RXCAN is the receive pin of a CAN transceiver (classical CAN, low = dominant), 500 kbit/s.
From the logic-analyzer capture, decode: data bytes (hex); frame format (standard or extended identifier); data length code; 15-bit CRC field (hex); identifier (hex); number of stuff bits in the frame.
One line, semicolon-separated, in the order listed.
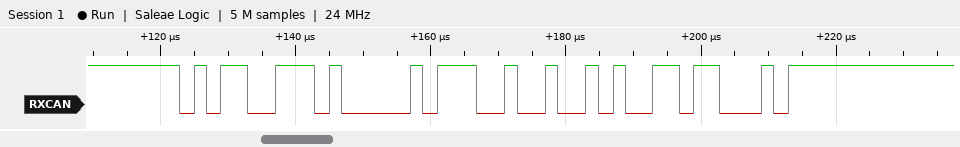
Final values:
C9; standard; 1; 0x14D8; 0x59D; 1
